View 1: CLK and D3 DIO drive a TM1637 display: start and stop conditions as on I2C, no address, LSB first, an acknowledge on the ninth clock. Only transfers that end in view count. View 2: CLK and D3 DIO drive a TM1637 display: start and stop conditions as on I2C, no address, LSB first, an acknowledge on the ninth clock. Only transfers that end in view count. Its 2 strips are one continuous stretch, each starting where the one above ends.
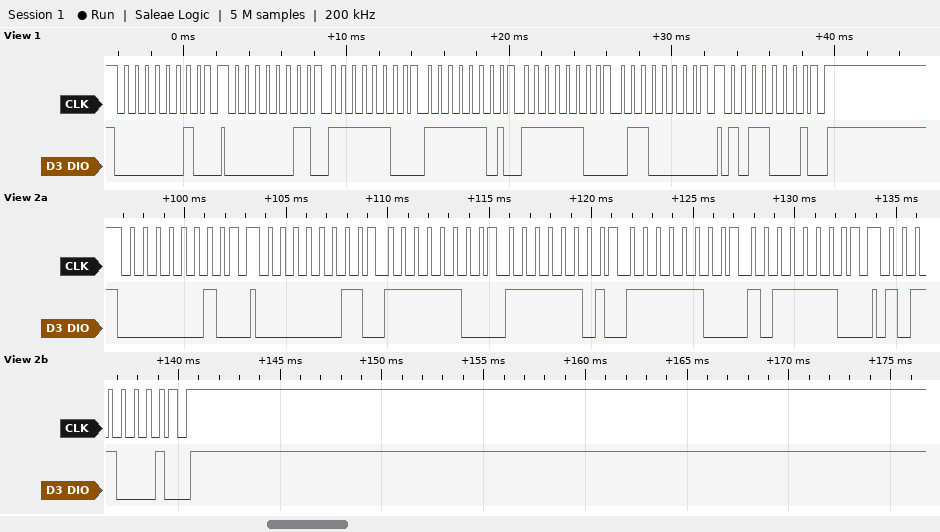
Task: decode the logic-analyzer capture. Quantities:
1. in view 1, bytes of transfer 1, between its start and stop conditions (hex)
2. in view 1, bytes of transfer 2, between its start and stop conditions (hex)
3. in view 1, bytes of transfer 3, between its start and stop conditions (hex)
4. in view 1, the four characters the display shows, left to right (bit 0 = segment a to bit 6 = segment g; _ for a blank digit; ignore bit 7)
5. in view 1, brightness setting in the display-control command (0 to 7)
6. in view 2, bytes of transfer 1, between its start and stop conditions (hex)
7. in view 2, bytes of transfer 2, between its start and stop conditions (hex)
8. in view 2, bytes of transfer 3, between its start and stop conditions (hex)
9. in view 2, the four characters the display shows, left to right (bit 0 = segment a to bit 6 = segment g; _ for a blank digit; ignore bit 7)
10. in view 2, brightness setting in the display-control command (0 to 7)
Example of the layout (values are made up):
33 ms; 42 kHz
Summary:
40; C0 3F BF 3F 06; 8D; 0001; 5; 40; C0 3F BF 3F 7D; 8D; 0006; 5
